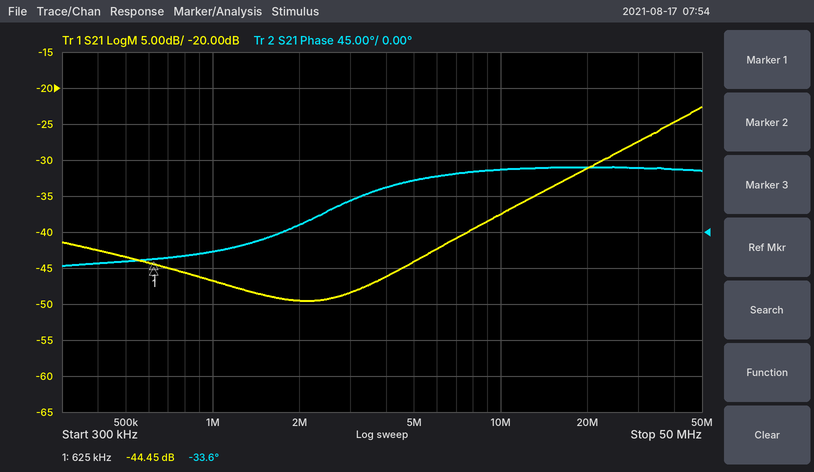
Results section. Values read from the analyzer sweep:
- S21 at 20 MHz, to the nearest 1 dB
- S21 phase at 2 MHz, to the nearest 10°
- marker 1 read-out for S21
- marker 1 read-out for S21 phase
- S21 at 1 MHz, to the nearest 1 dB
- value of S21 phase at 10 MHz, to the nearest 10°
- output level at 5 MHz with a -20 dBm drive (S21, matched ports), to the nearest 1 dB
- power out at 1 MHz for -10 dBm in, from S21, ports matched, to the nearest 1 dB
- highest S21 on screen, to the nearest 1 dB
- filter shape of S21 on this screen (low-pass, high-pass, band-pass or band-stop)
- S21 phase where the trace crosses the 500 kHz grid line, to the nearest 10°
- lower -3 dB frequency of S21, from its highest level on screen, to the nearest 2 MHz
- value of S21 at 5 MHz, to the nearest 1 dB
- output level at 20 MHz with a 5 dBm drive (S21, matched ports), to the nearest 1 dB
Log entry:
-31 dB
10°
-44.45 dB
-33.6°
-47 dB
80°
-64 dBm
-57 dBm
-23 dB
high-pass
-40°
36 MHz
-44 dB
-26 dBm
